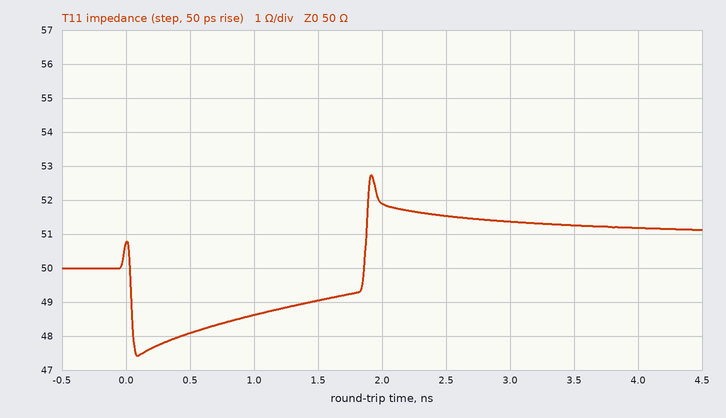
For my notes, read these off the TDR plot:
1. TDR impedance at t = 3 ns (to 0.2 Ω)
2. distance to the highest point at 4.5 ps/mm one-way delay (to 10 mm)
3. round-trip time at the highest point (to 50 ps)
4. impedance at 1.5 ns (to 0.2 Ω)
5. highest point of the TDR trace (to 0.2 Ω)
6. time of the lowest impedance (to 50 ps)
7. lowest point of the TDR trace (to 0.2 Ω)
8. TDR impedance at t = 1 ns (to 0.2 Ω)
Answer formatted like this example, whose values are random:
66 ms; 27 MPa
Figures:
51.4 Ω; 210 mm; 1.90 ns; 49.0 Ω; 52.8 Ω; 100 ps; 47.4 Ω; 48.6 Ω
